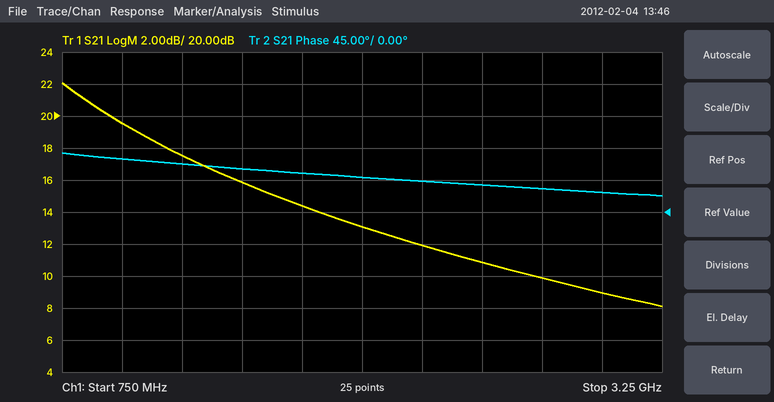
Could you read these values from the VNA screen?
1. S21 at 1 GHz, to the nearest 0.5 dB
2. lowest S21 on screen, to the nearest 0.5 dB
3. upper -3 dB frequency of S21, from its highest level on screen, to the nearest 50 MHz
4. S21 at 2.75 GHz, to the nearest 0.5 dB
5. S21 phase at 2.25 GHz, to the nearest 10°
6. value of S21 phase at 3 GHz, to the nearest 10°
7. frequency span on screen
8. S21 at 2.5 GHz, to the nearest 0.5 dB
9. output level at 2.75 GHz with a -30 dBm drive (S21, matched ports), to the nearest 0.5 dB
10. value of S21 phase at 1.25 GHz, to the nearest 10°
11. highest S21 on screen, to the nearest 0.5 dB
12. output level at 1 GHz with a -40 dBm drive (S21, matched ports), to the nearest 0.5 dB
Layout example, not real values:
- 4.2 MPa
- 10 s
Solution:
- 19.5 dB
- 8.0 dB
- 1.05 GHz
- 10.0 dB
- 40°
- 30°
- 2.5 GHz
- 11.0 dB
- -20.0 dBm
- 70°
- 22.0 dB
- -20.5 dBm
